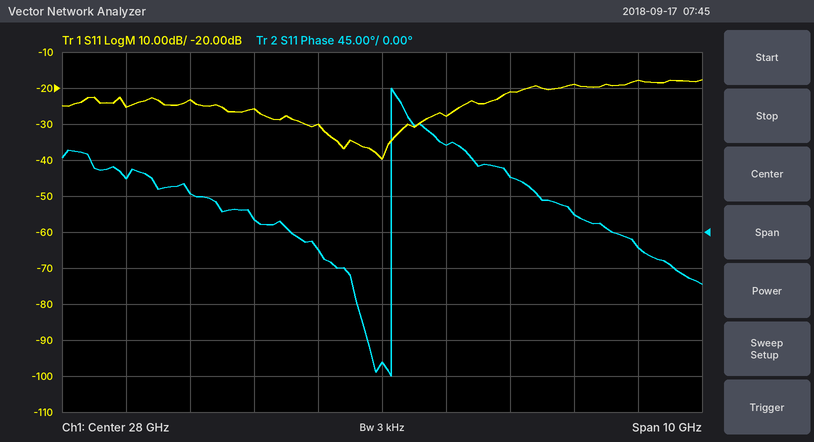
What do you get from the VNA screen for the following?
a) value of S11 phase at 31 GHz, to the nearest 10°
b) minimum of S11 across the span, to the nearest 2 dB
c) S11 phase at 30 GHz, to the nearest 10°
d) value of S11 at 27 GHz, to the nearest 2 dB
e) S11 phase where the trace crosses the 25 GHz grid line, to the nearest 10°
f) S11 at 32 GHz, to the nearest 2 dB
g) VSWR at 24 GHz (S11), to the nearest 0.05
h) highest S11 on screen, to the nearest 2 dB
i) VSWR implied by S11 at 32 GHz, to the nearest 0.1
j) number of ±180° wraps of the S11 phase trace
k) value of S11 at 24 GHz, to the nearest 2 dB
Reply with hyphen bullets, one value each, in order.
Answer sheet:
- 20°
- -40 dB
- 70°
- -30 dB
- 50°
- -18 dB
- 1.10
- -18 dB
- 1.3
- 1
- -26 dB
